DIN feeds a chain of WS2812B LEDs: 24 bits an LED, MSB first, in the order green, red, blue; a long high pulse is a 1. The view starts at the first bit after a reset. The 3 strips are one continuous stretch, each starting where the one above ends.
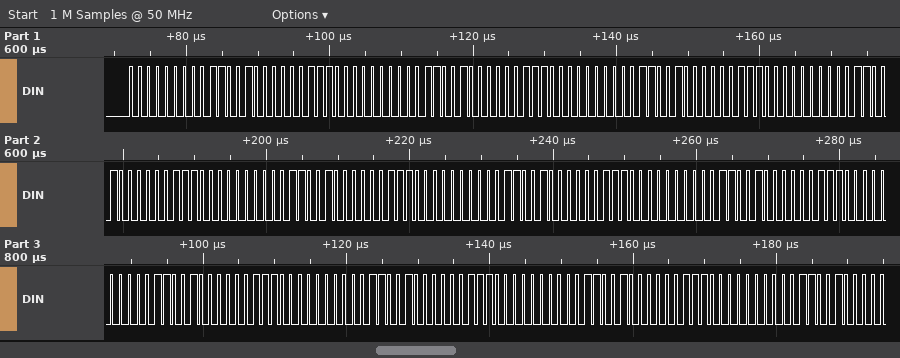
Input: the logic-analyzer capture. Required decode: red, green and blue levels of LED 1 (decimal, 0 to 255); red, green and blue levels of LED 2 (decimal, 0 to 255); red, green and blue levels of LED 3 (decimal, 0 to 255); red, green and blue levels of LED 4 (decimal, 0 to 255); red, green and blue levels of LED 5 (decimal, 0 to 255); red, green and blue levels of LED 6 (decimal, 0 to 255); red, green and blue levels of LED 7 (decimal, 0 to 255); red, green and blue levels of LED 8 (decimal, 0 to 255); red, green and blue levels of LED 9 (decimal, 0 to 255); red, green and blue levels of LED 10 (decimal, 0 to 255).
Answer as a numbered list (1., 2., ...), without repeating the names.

1. 100, 0, 14
2. 100, 0, 14
3. 100, 0, 14
4. 100, 0, 14
5. 100, 0, 14
6. 100, 0, 14
7. 100, 0, 14
8. 100, 0, 14
9. 100, 0, 14
10. 100, 0, 14
